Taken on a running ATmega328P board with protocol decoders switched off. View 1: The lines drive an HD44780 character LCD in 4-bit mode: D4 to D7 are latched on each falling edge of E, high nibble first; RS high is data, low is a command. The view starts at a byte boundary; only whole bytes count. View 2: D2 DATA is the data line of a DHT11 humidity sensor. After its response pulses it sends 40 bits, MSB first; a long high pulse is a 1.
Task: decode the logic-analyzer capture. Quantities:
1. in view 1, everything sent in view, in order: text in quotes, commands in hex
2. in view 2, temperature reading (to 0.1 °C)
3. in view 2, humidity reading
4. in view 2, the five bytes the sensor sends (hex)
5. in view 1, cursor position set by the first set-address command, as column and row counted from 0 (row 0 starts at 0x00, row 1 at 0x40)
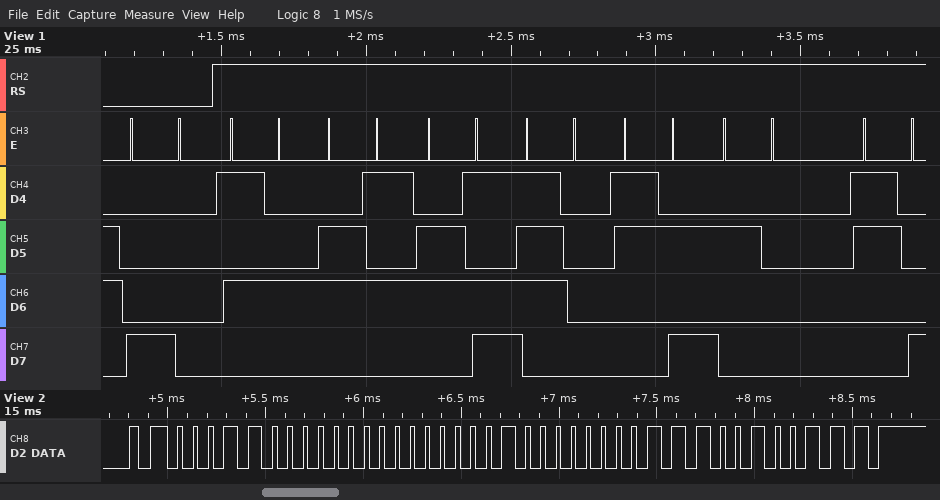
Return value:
0x80 "Temp: 8"
8.7 °C
24 %
18 00 08 07 27
column 0, row 0
